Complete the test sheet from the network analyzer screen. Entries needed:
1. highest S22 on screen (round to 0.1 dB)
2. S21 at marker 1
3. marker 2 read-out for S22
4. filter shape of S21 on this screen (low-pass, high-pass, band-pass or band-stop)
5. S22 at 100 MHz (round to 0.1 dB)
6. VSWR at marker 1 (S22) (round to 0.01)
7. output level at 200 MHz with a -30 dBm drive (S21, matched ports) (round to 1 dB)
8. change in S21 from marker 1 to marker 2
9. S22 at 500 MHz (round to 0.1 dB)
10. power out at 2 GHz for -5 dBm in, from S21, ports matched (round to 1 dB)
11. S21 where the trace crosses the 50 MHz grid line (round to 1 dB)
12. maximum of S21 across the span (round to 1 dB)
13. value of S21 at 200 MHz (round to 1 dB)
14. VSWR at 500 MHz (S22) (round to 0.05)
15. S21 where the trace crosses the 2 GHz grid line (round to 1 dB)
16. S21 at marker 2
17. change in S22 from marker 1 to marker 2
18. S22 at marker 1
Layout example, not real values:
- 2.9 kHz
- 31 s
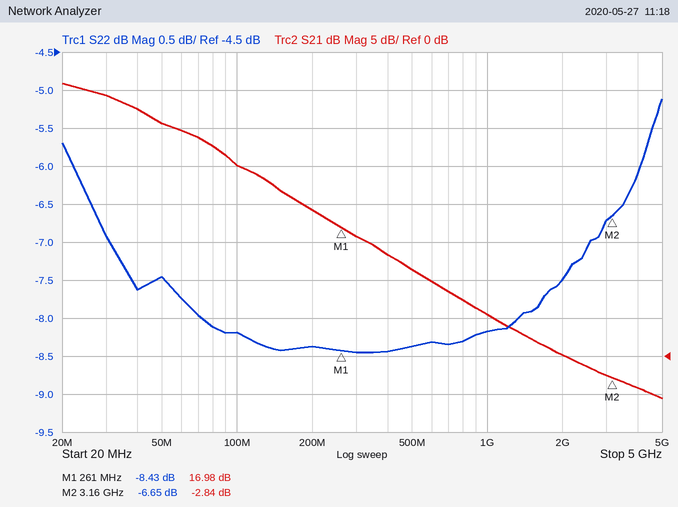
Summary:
- -5.1 dB
- 16.98 dB
- -6.65 dB
- low-pass
- -8.2 dB
- 2.22
- -11 dBm
- -19.82 dB
- -8.4 dB
- -5 dBm
- 31 dB
- 36 dB
- 19 dB
- 2.25
- 0 dB
- -2.84 dB
- 1.78 dB
- -8.43 dB
